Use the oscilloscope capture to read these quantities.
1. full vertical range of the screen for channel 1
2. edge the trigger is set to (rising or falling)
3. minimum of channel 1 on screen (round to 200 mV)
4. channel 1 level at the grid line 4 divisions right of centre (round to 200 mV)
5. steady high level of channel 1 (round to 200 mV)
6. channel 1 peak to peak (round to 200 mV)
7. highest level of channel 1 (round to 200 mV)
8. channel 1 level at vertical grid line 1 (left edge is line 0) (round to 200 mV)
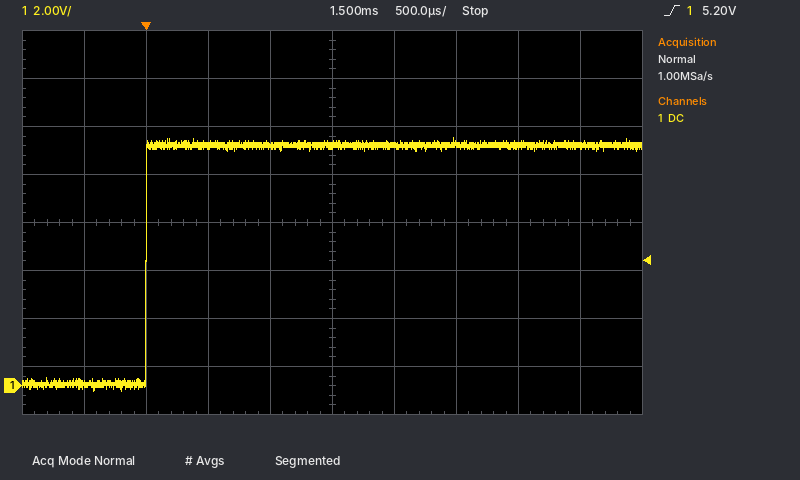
16 V
rising
-200 mV
10.0 V
10.0 V
10.6 V
10.4 V
0.0 V
